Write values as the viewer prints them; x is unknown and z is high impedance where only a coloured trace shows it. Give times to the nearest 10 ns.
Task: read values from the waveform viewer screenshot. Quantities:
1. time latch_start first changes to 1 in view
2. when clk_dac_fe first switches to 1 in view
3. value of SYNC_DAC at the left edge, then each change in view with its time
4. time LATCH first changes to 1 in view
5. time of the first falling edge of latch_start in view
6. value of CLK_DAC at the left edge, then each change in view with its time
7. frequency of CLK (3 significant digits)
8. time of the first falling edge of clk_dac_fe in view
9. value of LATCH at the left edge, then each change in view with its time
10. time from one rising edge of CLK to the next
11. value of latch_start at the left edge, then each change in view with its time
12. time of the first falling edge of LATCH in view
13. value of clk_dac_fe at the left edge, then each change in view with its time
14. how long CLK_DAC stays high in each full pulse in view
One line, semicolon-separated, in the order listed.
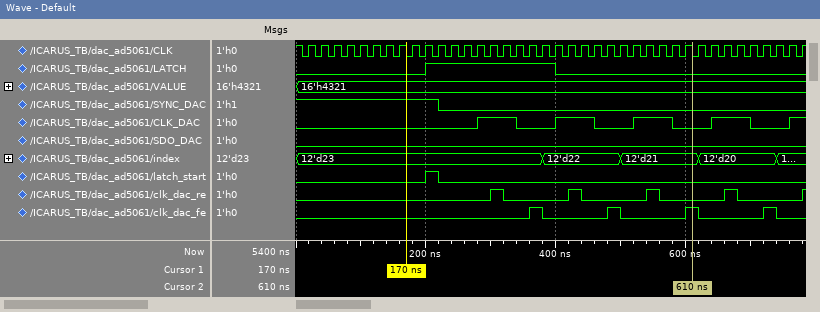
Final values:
200 ns; 360 ns; 1, 0 at 220 ns; 200 ns; 220 ns; 0, 1 at 280 ns, 0 at 340 ns, 1 at 400 ns, 0 at 460 ns, 1 at 520 ns, 0 at 580 ns, 1 at 640 ns, 0 at 700 ns, 1 at 760 ns; 50.0 MHz; 380 ns; 0, 1 at 200 ns, 0 at 400 ns; 20 ns; 0, 1 at 200 ns, 0 at 220 ns; 400 ns; 0, 1 at 360 ns, 0 at 380 ns, 1 at 480 ns, 0 at 500 ns, 1 at 600 ns, 0 at 620 ns, 1 at 720 ns, 0 at 740 ns; 60 ns, 60 ns, 60 ns, 60 ns
